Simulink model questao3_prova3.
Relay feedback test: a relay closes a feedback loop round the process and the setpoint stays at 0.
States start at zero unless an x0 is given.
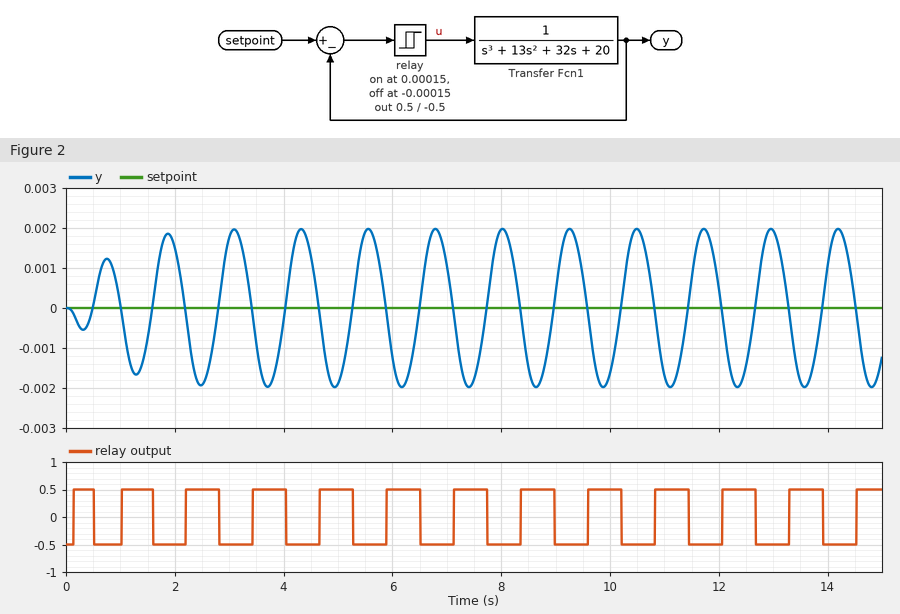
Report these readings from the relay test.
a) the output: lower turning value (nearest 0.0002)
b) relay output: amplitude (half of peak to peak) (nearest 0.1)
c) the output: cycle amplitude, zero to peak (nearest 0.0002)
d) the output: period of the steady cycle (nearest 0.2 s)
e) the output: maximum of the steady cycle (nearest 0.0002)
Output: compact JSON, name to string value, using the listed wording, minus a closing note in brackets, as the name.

{"the output: lower turning value": "-0.0020", "relay output: amplitude (half of peak to peak)": "0.5", "the output: cycle amplitude, zero to peak": "0.0020", "the output: period of the steady cycle": "1.2 s", "the output: maximum of the steady cycle": "0.0020"}
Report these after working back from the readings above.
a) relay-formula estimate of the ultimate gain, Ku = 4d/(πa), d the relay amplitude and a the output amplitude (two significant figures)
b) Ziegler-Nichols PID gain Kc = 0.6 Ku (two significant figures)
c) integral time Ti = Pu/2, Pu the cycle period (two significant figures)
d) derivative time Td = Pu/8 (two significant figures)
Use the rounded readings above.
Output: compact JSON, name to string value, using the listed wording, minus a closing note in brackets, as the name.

{"relay-formula estimate of the ultimate gain, Ku = 4d/(πa), d the relay amplitude and a the output amplitude": "320", "Ziegler-Nichols PID gain Kc = 0.6 Ku": "190", "integral time Ti = Pu/2, Pu the cycle period": "0.60 s", "derivative time Td = Pu/8": "0.15 s"}
